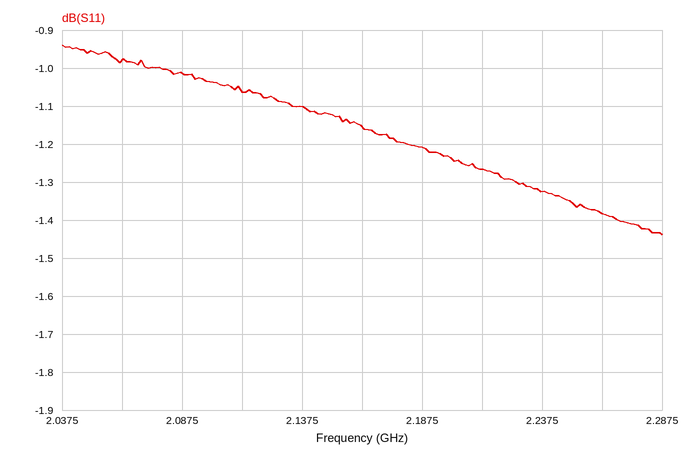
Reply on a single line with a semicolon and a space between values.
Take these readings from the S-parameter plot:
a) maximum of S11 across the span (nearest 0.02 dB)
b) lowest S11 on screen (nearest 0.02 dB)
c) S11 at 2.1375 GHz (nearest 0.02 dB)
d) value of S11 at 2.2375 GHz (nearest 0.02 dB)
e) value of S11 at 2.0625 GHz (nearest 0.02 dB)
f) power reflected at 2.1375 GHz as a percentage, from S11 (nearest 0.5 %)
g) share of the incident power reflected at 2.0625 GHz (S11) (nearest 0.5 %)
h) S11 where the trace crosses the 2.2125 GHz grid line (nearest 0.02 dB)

-0.94 dB; -1.44 dB; -1.10 dB; -1.32 dB; -0.98 dB; 77.5 %; 80.0 %; -1.26 dB
